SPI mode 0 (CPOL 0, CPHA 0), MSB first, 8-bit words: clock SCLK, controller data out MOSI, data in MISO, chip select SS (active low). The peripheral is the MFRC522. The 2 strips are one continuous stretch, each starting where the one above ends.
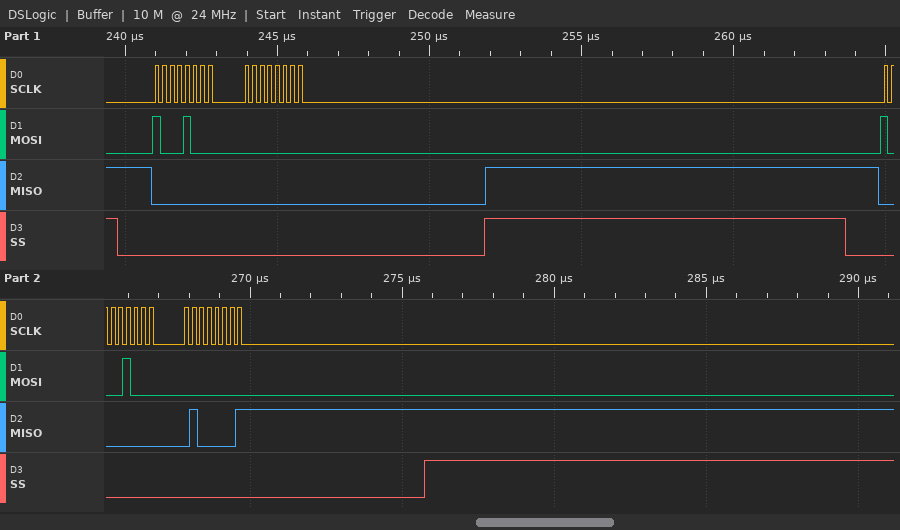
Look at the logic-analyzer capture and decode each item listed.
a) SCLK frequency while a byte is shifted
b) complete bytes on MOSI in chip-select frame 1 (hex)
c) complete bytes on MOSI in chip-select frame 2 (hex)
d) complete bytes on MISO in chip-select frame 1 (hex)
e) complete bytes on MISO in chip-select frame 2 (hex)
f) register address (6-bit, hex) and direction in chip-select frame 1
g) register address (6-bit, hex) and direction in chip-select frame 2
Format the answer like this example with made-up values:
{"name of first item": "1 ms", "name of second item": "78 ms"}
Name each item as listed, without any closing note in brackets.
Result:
{"SCLK frequency while a byte is shifted": "4 MHz", "complete bytes on MOSI in chip-select frame 1": "88 00", "complete bytes on MOSI in chip-select frame 2": "88 00", "complete bytes on MISO in chip-select frame 1": "00 00", "complete bytes on MISO in chip-select frame 2": "00 41", "register address (6-bit, hex) and direction in chip-select frame 1": "0x04 read", "register address (6-bit, hex) and direction in chip-select frame 2": "0x04 read"}
